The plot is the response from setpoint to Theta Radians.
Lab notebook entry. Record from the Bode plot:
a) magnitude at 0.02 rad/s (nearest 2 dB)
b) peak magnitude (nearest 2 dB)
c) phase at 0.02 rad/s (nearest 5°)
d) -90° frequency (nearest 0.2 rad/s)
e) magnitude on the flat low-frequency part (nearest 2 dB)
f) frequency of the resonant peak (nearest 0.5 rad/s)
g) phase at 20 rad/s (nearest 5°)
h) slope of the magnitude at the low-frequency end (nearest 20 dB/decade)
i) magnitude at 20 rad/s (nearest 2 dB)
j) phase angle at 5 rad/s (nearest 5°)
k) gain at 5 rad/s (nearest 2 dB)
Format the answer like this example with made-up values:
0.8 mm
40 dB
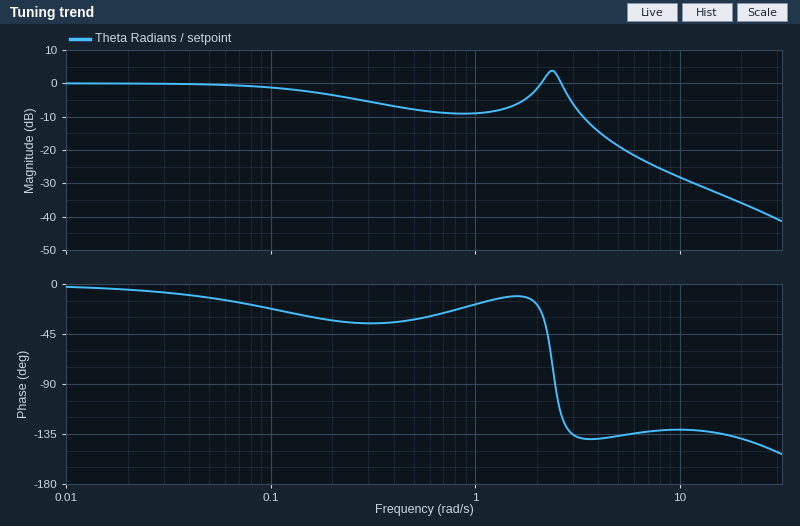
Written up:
0 dB
4 dB
-5°
2.4 rad/s
0 dB
2.5 rad/s
-140°
0 dB/decade
-36 dB
-135°
-18 dB
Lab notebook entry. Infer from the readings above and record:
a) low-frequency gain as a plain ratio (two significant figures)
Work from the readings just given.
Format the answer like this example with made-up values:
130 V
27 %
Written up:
1.0
